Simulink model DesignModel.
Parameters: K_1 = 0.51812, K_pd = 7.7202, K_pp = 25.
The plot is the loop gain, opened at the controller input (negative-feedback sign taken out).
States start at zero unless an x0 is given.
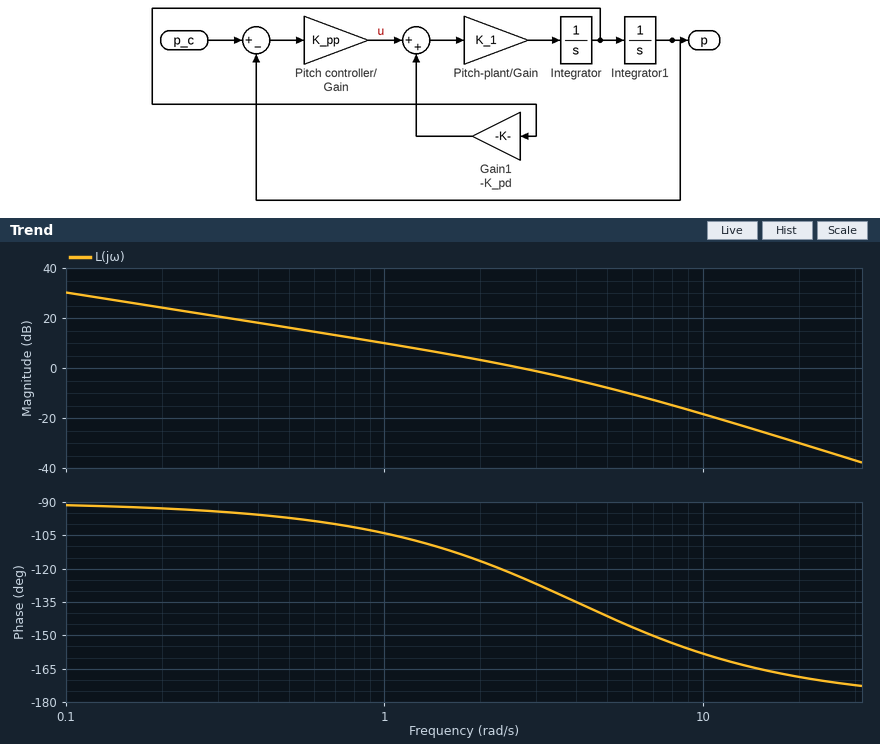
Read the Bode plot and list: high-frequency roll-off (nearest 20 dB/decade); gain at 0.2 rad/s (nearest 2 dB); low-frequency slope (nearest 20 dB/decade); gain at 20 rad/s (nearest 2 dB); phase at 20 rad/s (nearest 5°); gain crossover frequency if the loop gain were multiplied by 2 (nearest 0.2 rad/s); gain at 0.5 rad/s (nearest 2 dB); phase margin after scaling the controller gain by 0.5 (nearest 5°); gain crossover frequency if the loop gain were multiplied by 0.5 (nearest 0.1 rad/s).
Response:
-40 dB/decade
24 dB
-20 dB/decade
-30 dB
-170°
4.4 rad/s
16 dB
70°
1.5 rad/s
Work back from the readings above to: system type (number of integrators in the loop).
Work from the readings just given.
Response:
1
